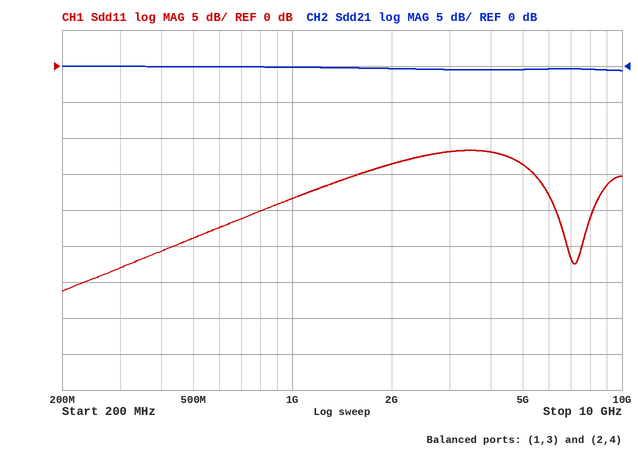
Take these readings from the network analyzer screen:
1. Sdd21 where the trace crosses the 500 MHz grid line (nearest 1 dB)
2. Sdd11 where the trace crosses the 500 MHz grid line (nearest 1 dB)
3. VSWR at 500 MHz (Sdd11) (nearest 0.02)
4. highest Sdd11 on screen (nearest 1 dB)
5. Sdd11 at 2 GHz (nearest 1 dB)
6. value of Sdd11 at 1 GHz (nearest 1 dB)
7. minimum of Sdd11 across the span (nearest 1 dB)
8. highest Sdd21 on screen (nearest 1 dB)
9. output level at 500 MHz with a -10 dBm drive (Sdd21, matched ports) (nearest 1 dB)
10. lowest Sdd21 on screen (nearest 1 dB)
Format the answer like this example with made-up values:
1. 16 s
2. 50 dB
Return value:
1. 0 dB
2. -24 dB
3. 1.14
4. -12 dB
5. -14 dB
6. -18 dB
7. -31 dB
8. 0 dB
9. -10 dBm
10. -1 dB
